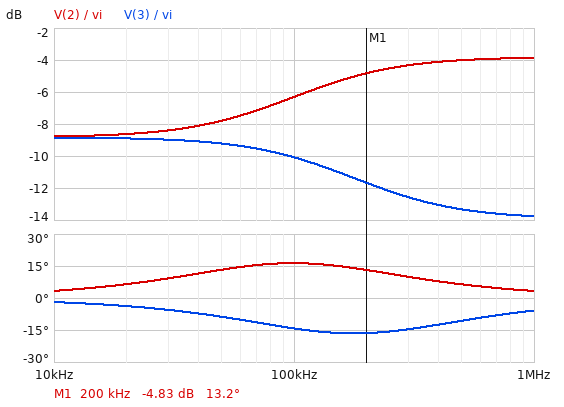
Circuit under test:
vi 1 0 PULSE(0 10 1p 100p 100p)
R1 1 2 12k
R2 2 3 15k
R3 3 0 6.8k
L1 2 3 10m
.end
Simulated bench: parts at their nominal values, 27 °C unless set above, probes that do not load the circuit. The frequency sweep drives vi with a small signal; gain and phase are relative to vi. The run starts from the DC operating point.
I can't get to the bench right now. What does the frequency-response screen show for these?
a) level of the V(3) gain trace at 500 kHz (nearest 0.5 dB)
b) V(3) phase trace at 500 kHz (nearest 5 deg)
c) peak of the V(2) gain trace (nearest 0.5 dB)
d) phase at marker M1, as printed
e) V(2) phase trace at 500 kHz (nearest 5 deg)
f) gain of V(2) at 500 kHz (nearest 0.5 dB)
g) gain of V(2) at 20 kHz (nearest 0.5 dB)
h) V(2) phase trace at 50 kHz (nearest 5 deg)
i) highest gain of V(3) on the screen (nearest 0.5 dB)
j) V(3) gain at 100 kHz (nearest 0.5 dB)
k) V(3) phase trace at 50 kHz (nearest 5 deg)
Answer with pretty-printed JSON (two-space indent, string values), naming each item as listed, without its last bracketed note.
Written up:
{
  "level of the V(3) gain trace at 500 kHz": "-13.5 dB",
  "V(3) phase trace at 500 kHz": "-10 deg",
  "peak of the V(2) gain trace": "-4.0 dB",
  "phase at marker M1, as printed": "13.2 deg",
  "V(2) phase trace at 500 kHz": "5 deg",
  "gain of V(2) at 500 kHz": "-4.0 dB",
  "gain of V(2) at 20 kHz": "-8.5 dB",
  "V(2) phase trace at 50 kHz": "15 deg",
  "highest gain of V(3) on the screen": "-9.0 dB",
  "V(3) gain at 100 kHz": "-10.0 dB",
  "V(3) phase trace at 50 kHz": "-10 deg"
}
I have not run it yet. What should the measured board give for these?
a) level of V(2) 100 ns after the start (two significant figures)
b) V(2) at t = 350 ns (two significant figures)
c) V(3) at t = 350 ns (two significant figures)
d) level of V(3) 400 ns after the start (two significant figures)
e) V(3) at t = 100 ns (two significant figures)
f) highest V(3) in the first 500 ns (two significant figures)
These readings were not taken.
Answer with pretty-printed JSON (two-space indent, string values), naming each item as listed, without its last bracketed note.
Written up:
{
  "level of V(2) 100 ns after the start": "6.2 V",
  "V(2) at t = 350 ns": "5.7 V",
  "V(3) at t = 350 ns": "2.4 V",
  "level of V(3) 400 ns after the start": "2.5 V",
  "V(3) at t = 100 ns": "2.1 V",
  "highest V(3) in the first 500 ns": "2.6 V"
}
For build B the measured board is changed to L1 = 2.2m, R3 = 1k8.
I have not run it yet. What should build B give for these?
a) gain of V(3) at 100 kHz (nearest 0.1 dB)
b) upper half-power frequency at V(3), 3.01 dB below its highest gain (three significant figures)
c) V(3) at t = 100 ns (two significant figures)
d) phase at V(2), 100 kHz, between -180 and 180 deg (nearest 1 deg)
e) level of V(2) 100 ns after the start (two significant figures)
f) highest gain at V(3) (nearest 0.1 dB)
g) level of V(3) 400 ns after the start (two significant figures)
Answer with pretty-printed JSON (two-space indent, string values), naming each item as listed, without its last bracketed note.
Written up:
{
  "gain of V(3) at 100 kHz": "-17.8 dB",
  "upper half-power frequency at V(3), 3.01 dB below its highest gain": "707 kHz",
  "V(3) at t = 100 ns": "810 mV",
  "phase at V(2), 100 kHz, between -180 and 180 deg": "30 deg",
  "level of V(2) 100 ns after the start": "4.6 V",
  "highest gain at V(3)": "-17.7 dB",
  "level of V(3) 400 ns after the start": "1.1 V"
}
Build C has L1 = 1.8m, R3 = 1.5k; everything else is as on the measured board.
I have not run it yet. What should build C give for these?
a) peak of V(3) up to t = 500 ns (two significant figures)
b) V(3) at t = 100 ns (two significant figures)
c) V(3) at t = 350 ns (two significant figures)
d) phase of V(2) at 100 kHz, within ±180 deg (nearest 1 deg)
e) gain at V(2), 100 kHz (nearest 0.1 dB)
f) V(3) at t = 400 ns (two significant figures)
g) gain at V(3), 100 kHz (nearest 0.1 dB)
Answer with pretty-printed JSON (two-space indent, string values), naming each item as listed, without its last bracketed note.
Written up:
{
  "peak of V(3) up to t = 500 ns": "1.0 V",
  "V(3) at t = 100 ns": "720 mV",
  "V(3) at t = 350 ns": "960 mV",
  "phase of V(2) at 100 kHz, within ±180 deg": "31 deg",
  "gain at V(2), 100 kHz": "-16.9 dB",
  "V(3) at t = 400 ns": "990 mV",
  "gain at V(3), 100 kHz": "-19.2 dB"
}
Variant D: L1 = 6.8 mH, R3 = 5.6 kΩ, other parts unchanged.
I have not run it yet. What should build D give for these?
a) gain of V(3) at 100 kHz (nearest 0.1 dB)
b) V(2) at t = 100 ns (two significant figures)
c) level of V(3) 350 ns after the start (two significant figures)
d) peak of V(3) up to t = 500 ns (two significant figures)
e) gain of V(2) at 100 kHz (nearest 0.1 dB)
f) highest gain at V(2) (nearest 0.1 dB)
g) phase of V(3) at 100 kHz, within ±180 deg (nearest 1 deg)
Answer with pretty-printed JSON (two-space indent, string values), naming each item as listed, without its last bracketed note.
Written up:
{
  "gain of V(3) at 100 kHz": "-10.7 dB",
  "V(2) at t = 100 ns": "6.0 V",
  "level of V(3) 350 ns after the start": "2.2 V",
  "peak of V(3) up to t = 500 ns": "2.4 V",
  "gain of V(2) at 100 kHz": "-7.8 dB",
  "highest gain at V(2)": "-4.0 dB",
  "phase of V(3) at 100 kHz, within ±180 deg": "-12 deg"
}
